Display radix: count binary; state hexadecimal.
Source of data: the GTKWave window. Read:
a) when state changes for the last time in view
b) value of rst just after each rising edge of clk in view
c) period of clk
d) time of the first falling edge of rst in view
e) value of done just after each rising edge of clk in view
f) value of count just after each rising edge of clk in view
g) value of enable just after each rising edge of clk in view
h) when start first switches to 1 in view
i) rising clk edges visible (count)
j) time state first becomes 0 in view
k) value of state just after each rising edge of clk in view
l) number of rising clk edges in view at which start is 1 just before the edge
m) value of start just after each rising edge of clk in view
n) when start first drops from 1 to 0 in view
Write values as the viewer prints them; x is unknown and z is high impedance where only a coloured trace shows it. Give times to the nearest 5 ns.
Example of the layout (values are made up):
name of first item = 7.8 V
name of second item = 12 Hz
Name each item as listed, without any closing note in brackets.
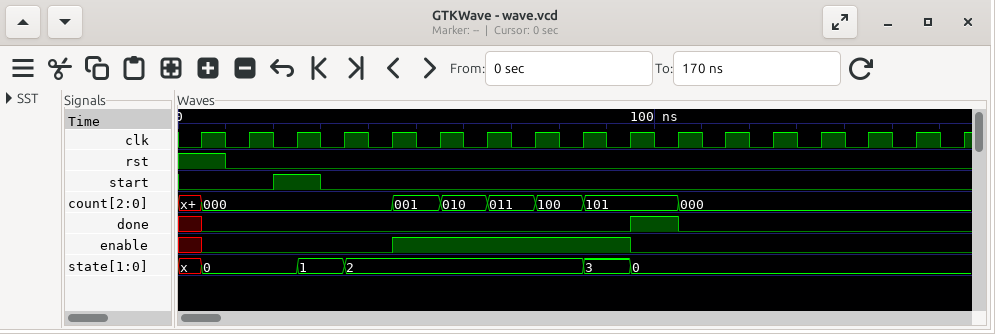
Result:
when state changes for the last time in view = 95 ns
value of rst just after each rising edge of clk in view = 1 0 0 0 0 0 0 0 0 0 0 0 0 0 0 0 0
period of clk = 10 ns
time of the first falling edge of rst in view = 10 ns
value of done just after each rising edge of clk in view = 0 0 0 0 0 0 0 0 0 1 0 0 0 0 0 0 0
value of count just after each rising edge of clk in view = 000, 000, 000, 000, 001, 010, 011, 100, 101, 101, 000, 000, 000, 000, 000, 000, 000
value of enable just after each rising edge of clk in view = 0 0 0 0 1 1 1 1 1 0 0 0 0 0 0 0 0
when start first switches to 1 in view = 20 ns
rising clk edges visible = 17
time state first becomes 0 in view = 5 ns
value of state just after each rising edge of clk in view = 0, 0, 1, 2, 2, 2, 2, 2, 3, 0, 0, 0, 0, 0, 0, 0, 0
number of rising clk edges in view at which start is 1 just before the edge = 1
value of start just after each rising edge of clk in view = 0 0 1 0 0 0 0 0 0 0 0 0 0 0 0 0 0
when start first drops from 1 to 0 in view = 30 ns
